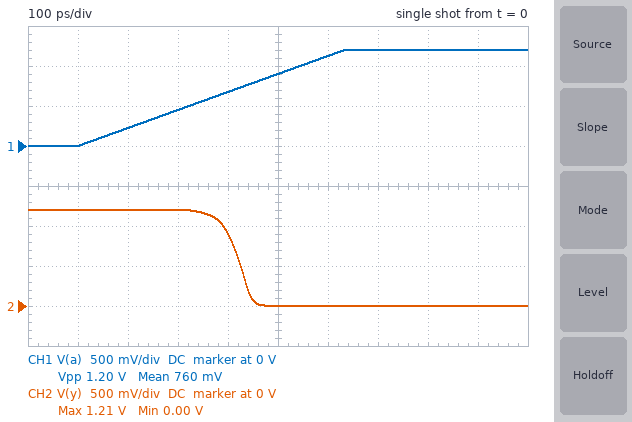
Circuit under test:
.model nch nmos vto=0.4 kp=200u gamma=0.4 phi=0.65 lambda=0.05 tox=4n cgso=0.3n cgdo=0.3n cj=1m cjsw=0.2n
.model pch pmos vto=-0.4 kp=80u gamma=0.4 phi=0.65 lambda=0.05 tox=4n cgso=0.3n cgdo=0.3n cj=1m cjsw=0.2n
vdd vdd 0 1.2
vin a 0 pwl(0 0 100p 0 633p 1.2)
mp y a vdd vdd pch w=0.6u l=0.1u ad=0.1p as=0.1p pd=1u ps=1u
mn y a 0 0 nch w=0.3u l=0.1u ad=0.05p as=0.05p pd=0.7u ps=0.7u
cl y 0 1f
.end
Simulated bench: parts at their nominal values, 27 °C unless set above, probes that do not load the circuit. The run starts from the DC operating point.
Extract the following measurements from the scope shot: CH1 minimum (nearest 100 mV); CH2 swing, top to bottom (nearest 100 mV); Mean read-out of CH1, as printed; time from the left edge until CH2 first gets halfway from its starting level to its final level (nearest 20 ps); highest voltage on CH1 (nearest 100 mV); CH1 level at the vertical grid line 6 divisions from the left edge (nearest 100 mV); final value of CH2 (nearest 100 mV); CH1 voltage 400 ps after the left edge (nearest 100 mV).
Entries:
0 V
1.2 V
760 mV
420 ps
1.2 V
1.1 V
0 V
700 mV
